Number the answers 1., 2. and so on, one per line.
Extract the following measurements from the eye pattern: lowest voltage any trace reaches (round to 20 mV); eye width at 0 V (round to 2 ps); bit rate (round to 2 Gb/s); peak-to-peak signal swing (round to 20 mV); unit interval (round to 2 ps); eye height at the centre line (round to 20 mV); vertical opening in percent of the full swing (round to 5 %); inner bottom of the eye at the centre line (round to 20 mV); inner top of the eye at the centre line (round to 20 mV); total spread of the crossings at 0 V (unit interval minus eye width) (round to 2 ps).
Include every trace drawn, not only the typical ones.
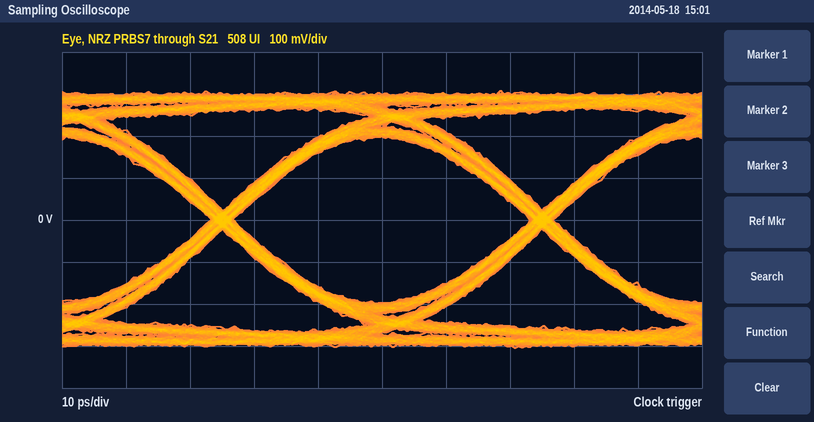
1. -300 mV
2. 46 ps
3. 20 Gb/s
4. 620 mV
5. 50 ps
6. 400 mV
7. 65 %
8. -200 mV
9. 200 mV
10. 4 ps
